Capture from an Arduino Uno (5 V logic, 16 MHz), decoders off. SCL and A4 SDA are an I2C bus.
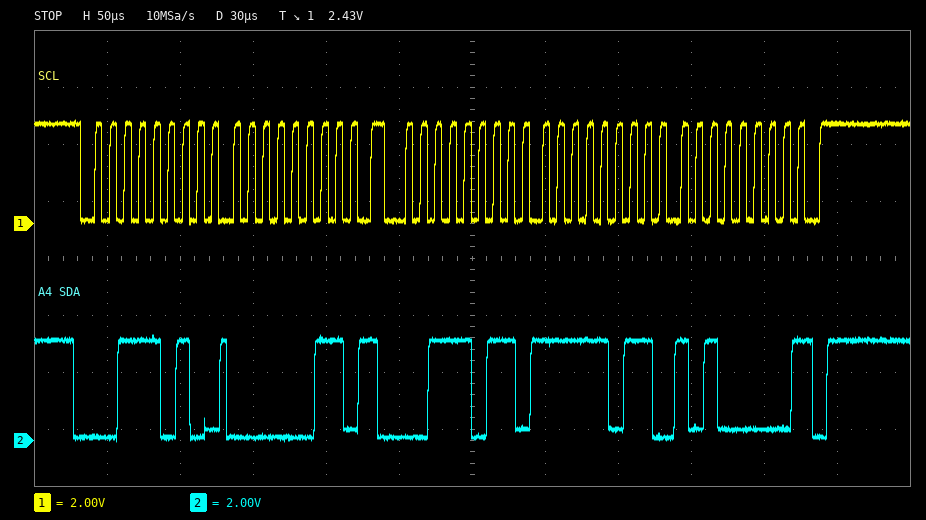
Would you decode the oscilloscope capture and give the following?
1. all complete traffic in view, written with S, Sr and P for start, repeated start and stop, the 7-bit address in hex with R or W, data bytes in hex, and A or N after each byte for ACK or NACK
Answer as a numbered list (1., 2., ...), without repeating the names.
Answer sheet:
1. S 1DW A 03 A Sr 1DR A FB A A0 N P
